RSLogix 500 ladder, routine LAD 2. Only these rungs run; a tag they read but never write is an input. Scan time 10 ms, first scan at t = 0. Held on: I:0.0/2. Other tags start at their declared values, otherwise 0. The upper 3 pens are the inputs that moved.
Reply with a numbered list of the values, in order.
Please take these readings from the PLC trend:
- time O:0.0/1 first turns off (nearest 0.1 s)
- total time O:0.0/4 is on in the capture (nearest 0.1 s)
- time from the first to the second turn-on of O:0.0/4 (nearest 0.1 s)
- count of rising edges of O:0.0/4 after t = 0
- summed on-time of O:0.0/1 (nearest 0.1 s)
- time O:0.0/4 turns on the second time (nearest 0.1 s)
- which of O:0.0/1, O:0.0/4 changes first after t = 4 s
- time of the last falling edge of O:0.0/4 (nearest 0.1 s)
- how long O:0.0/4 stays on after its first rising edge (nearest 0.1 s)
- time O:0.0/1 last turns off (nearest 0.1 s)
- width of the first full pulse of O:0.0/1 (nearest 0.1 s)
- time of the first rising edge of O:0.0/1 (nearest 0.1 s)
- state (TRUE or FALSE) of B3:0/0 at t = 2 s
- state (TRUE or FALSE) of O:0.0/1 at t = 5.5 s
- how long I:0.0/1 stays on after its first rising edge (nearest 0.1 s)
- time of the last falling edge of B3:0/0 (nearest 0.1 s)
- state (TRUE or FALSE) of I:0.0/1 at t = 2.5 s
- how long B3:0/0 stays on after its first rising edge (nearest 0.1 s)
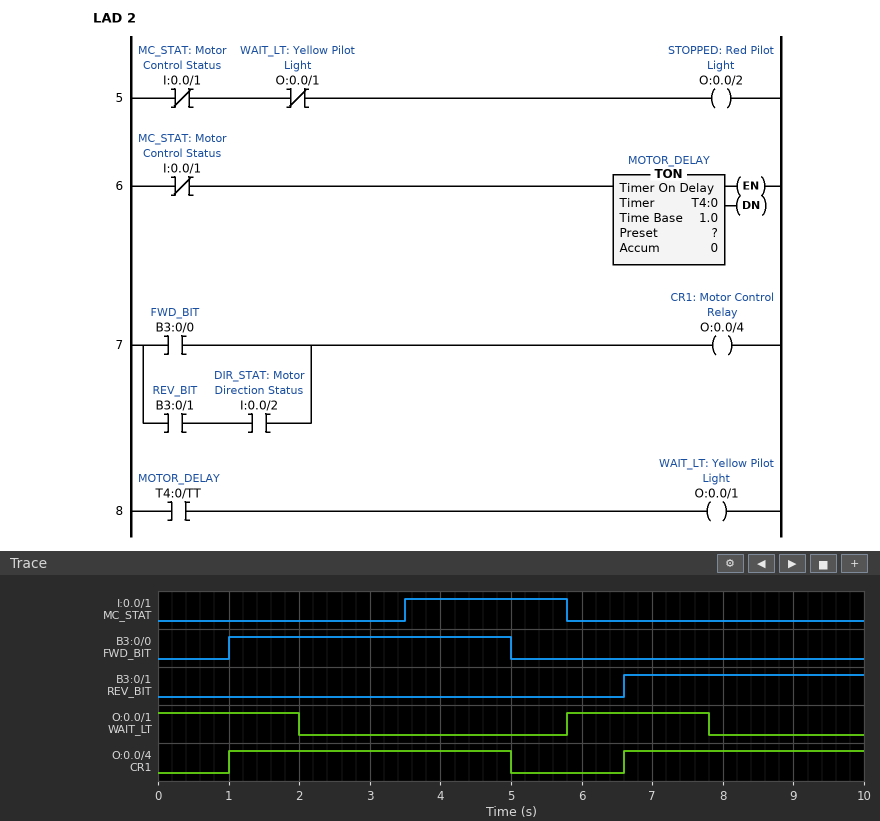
1. 2.0 s
2. 7.4 s
3. 5.6 s
4. 2
5. 4.0 s
6. 6.6 s
7. O:0.0/4
8. 5.0 s
9. 4.0 s
10. 7.8 s
11. 2.0 s
12. 5.8 s
13. TRUE
14. FALSE
15. 2.3 s
16. 5.0 s
17. FALSE
18. 4.0 s
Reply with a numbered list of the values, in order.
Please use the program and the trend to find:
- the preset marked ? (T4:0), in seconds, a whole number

1. 2 s
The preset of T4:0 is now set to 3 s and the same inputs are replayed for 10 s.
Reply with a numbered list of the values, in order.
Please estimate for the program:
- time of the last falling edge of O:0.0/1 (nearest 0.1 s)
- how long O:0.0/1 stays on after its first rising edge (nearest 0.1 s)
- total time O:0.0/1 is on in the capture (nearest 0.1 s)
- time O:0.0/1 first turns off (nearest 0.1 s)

1. 8.8 s
2. 3.0 s
3. 6.0 s
4. 3.0 s
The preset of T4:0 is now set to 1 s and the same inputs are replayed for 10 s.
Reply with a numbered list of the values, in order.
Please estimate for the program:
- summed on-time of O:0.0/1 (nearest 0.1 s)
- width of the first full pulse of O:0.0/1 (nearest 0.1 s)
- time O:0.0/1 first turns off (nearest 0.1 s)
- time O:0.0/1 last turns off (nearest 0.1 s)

1. 2.0 s
2. 1.0 s
3. 1.0 s
4. 6.8 s
